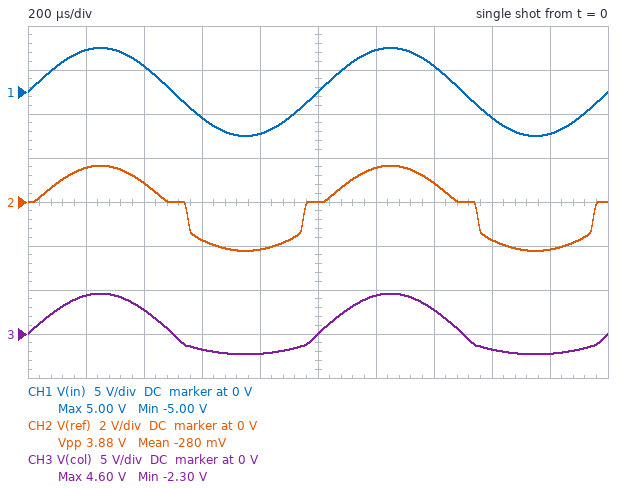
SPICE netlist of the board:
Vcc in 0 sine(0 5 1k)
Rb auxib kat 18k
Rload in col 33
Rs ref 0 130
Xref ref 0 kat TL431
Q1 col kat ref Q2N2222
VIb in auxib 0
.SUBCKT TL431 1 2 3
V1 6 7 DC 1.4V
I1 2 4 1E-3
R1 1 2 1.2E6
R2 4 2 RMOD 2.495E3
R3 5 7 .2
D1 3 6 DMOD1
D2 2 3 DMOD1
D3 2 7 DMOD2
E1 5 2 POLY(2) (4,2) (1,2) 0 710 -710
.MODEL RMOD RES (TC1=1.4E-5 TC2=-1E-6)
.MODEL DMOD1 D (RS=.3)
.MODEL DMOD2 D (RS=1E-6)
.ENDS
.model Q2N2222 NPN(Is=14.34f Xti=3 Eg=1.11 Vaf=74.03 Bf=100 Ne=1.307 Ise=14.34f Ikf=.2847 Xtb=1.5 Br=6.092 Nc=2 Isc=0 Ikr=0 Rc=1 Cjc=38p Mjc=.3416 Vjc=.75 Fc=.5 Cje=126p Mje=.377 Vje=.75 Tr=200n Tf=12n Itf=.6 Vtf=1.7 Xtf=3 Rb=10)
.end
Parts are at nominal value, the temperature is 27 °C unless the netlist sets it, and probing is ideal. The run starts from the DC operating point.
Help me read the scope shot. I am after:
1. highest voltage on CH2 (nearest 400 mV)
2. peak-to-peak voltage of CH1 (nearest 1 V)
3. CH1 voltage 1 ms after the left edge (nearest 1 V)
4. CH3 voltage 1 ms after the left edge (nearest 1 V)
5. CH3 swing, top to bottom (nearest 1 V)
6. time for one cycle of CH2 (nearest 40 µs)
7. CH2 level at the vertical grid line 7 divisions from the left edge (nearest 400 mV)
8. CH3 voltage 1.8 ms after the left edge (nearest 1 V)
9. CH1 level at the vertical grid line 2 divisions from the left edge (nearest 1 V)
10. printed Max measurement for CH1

1.6 V
10 V
0 V
0 V
7 V
1.00 ms
800 mV
-2 V
3 V
5.00 V
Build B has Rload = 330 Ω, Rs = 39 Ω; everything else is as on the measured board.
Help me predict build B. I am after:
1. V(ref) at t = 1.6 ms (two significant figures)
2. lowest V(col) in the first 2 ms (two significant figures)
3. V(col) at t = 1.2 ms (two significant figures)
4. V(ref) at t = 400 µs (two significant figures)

-160 mV
-1.4 V
610 mV
300 mV
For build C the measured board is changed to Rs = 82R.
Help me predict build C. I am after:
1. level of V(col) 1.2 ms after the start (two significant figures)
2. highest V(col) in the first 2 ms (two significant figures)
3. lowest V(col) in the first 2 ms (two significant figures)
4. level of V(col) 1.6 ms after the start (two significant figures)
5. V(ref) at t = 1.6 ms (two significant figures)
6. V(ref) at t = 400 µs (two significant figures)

4.3 V
4.5 V
-2.2 V
-1.7 V
-1.7 V
630 mV
